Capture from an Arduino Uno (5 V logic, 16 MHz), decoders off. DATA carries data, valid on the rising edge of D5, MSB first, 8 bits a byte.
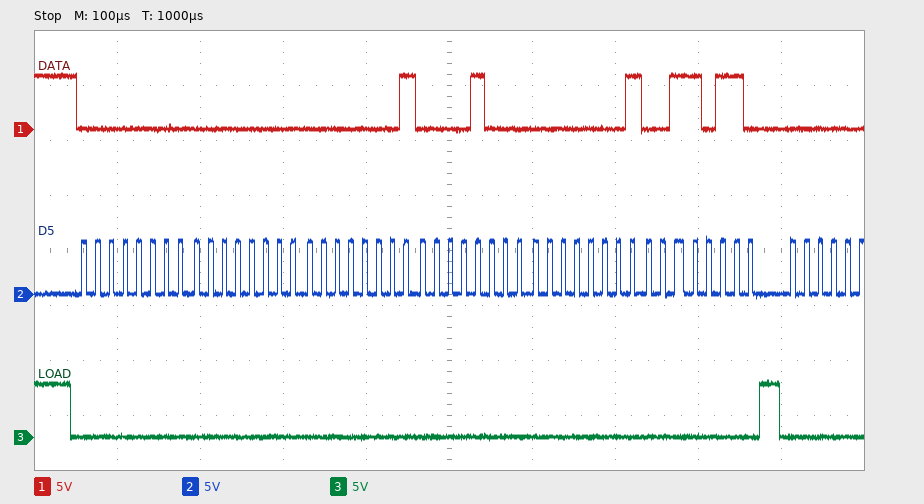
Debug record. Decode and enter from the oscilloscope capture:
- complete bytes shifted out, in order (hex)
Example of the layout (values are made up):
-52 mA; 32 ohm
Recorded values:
00 00 01 08 01 36
